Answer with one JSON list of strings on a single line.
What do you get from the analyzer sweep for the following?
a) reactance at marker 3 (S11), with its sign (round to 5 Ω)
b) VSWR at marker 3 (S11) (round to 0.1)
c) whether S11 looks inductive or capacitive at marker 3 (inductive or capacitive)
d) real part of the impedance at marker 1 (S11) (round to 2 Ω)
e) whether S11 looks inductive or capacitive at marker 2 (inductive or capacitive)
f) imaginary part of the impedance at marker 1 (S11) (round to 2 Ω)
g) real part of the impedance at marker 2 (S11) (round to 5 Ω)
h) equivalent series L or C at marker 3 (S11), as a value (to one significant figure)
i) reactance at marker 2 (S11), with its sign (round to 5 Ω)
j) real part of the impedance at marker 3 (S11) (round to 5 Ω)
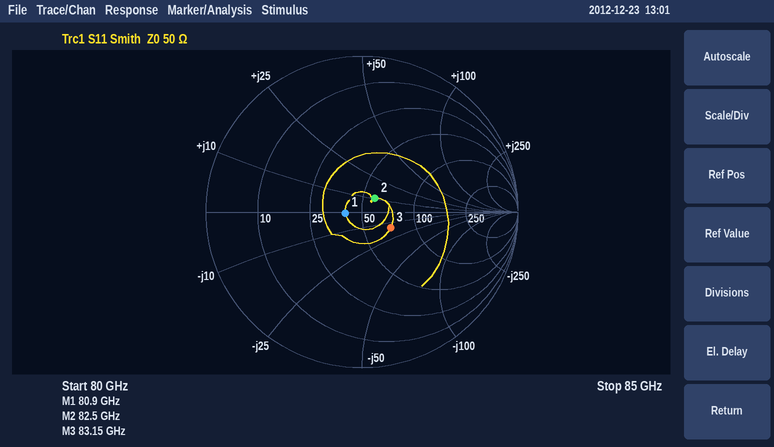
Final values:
["-15 Ω", "1.5", "capacitive", "40 Ω", "inductive", "0 Ω", "60 Ω", "100 fF", "+10 Ω", "70 Ω"]
